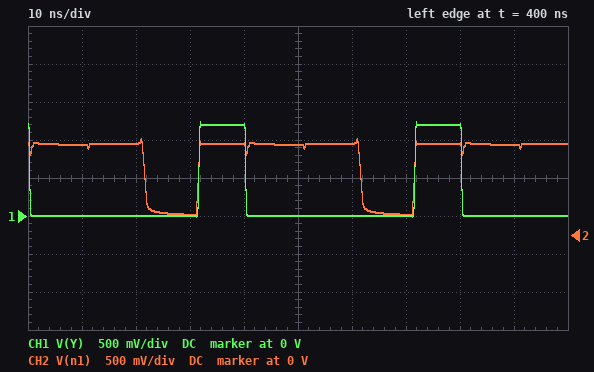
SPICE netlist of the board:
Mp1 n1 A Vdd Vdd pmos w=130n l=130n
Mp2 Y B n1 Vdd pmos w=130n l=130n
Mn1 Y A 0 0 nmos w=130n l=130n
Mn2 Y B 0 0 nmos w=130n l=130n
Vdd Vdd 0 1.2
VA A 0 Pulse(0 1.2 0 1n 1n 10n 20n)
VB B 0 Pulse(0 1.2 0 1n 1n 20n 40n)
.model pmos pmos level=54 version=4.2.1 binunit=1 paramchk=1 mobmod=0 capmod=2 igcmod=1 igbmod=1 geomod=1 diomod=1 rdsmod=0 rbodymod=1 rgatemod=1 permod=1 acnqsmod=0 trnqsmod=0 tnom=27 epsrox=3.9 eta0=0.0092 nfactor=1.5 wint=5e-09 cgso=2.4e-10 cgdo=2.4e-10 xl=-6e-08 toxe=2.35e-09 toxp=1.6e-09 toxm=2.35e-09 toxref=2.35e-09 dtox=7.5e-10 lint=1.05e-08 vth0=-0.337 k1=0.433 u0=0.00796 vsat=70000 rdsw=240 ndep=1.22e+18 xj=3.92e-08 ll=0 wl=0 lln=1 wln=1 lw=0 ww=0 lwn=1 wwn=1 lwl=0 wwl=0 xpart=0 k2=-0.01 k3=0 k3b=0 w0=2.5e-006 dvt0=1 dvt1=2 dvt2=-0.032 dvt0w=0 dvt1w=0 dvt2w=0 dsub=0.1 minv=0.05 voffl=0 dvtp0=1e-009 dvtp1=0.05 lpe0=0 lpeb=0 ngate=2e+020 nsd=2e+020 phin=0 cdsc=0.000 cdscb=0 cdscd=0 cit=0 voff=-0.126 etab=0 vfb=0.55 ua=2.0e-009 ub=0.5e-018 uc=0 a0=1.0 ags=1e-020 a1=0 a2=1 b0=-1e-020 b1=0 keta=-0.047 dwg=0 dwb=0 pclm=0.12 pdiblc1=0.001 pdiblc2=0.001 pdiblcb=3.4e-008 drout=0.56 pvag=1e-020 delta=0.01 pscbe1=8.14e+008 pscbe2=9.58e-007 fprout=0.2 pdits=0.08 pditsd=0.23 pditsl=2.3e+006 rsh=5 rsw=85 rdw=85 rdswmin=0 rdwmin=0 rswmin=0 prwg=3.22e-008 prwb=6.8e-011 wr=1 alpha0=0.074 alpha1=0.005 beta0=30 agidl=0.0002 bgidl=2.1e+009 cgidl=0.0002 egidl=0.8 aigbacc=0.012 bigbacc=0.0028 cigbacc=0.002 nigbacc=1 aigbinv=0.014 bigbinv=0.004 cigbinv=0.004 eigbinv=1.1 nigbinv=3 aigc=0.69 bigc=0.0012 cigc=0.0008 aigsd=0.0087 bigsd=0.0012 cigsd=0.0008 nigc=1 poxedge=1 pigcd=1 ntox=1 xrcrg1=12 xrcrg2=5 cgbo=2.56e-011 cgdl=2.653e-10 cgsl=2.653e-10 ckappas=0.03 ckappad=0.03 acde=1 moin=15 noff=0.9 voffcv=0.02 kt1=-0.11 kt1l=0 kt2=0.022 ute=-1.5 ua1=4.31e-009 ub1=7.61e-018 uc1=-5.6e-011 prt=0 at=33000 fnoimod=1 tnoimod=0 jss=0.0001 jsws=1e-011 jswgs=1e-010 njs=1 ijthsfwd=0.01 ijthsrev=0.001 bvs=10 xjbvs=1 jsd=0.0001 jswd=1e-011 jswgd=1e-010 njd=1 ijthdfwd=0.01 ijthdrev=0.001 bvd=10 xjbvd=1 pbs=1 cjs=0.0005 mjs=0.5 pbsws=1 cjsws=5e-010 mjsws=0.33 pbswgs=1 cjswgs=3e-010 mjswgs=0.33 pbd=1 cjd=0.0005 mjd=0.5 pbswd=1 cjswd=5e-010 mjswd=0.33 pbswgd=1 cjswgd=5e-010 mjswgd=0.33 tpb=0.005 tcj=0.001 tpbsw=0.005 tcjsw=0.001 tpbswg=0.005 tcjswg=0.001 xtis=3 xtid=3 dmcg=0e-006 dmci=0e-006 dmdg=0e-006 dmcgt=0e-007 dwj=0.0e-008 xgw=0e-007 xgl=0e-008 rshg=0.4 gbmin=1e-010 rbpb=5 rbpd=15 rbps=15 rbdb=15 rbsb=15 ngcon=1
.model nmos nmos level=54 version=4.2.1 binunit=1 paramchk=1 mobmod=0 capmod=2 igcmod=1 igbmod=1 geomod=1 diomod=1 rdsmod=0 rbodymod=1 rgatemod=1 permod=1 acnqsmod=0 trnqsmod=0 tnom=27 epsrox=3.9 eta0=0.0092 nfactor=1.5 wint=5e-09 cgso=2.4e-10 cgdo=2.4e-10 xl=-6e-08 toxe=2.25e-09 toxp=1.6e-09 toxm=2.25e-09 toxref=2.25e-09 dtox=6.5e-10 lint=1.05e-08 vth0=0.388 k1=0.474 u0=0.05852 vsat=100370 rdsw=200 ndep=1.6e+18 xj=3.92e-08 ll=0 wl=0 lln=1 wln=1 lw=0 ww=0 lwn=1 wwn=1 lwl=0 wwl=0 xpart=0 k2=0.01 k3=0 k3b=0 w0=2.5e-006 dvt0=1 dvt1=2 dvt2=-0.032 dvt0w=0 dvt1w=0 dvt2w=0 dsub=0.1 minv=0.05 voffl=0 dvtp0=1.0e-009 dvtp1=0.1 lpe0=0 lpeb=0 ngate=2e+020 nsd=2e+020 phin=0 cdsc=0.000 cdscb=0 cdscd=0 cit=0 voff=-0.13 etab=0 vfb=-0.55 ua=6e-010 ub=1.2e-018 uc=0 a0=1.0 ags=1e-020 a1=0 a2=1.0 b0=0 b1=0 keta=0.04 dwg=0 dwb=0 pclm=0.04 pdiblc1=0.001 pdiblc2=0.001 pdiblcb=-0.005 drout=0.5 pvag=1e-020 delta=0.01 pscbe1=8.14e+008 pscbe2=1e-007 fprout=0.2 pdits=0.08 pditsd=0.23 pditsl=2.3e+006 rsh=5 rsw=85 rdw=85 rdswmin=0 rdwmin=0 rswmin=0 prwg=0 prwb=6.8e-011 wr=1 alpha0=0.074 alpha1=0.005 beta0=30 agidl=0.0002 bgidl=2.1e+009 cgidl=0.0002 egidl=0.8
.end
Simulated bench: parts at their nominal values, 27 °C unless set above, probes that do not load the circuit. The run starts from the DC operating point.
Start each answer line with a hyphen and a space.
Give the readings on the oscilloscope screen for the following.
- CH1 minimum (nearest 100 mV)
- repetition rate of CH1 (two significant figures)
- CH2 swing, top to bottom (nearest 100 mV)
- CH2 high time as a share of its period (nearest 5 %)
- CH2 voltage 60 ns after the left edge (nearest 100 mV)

- 0 V
- 25 MHz
- 1.0 V
- 75 %
- 1.2 V
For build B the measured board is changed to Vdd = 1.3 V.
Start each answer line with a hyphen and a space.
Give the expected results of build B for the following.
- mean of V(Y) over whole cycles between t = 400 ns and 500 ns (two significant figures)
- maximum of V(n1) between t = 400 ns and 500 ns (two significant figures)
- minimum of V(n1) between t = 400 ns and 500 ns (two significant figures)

- 280 mV
- 1.3 V
- 330 mV
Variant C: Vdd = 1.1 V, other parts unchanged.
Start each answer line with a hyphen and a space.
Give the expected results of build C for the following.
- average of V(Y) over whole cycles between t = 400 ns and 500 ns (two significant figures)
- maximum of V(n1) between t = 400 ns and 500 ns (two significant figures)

- 240 mV
- 1.2 V
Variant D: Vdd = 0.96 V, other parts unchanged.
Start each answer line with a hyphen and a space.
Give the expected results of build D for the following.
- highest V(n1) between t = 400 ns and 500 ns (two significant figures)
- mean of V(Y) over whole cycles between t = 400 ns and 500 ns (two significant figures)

- 1.1 V
- 210 mV
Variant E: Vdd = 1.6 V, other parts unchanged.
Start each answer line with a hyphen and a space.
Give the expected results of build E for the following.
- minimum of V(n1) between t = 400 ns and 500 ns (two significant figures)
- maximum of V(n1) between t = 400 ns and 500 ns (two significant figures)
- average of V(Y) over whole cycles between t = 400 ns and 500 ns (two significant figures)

- 620 mV
- 1.6 V
- 360 mV
